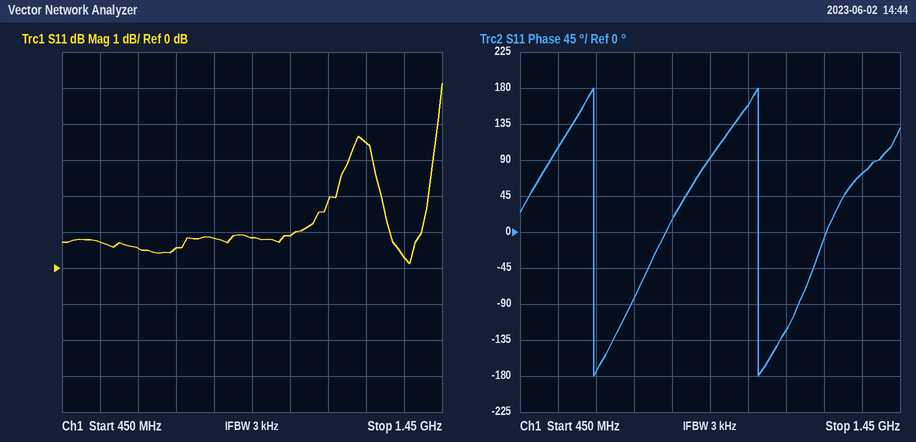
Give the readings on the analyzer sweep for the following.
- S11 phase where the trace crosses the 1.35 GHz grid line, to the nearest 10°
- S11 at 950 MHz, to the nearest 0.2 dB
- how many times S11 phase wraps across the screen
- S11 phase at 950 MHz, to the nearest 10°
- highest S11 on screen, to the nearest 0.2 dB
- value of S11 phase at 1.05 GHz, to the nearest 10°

70°
0.8 dB
2
90°
5.2 dB
160°
